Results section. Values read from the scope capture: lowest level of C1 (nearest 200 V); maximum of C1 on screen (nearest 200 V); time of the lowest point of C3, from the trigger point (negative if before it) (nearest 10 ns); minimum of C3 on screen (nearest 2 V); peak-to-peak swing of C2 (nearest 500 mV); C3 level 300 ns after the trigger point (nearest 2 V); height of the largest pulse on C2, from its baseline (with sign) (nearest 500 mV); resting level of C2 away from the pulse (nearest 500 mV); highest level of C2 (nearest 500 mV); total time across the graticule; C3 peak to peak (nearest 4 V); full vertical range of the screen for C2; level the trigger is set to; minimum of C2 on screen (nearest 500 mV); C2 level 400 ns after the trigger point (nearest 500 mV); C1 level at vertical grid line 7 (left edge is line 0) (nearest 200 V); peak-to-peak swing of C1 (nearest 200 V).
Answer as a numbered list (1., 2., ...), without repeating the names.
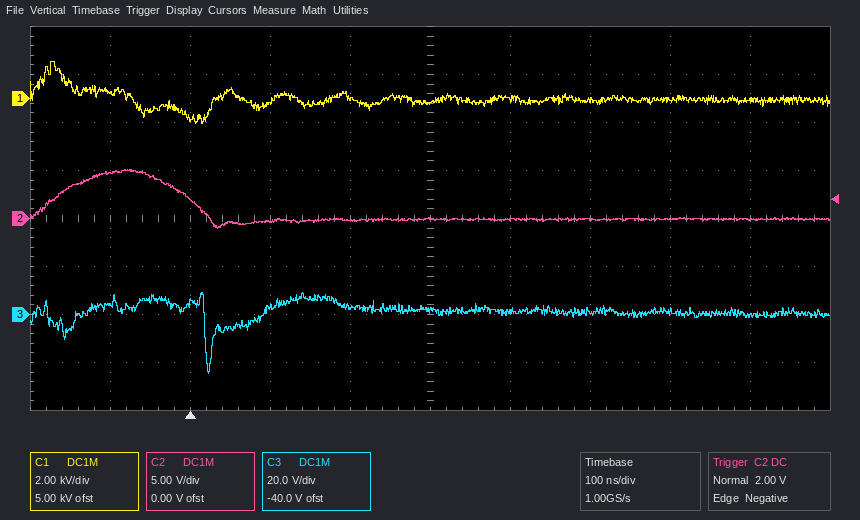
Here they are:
1. -1.0 kV
2. 1.6 kV
3. +20 ns
4. -24 V
5. 6.0 V
6. 2 V
7. +5.0 V
8. 0.0 V
9. 5.0 V
10. 1 µs
11. 32 V
12. 40 V
13. 2.00 V
14. -1.0 V
15. 0.0 V
16. 0.0 kV
17. 2.6 kV
